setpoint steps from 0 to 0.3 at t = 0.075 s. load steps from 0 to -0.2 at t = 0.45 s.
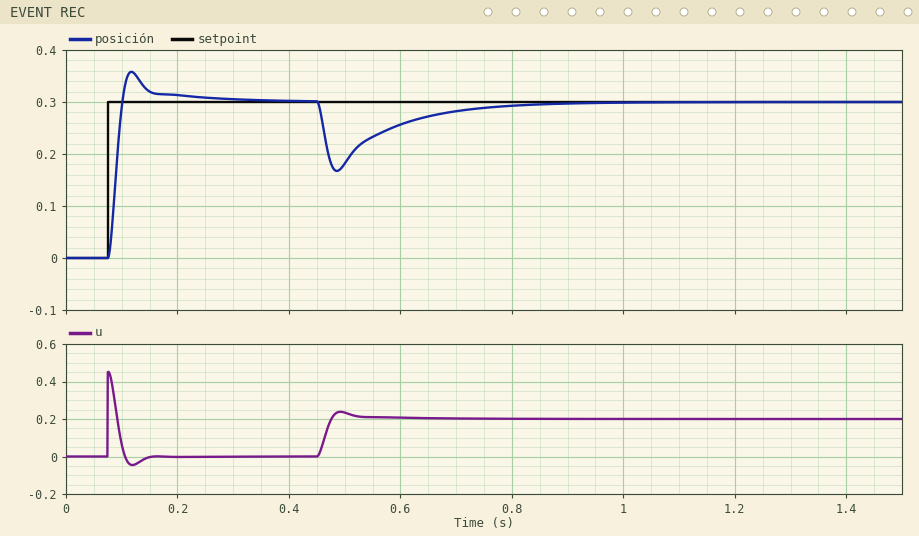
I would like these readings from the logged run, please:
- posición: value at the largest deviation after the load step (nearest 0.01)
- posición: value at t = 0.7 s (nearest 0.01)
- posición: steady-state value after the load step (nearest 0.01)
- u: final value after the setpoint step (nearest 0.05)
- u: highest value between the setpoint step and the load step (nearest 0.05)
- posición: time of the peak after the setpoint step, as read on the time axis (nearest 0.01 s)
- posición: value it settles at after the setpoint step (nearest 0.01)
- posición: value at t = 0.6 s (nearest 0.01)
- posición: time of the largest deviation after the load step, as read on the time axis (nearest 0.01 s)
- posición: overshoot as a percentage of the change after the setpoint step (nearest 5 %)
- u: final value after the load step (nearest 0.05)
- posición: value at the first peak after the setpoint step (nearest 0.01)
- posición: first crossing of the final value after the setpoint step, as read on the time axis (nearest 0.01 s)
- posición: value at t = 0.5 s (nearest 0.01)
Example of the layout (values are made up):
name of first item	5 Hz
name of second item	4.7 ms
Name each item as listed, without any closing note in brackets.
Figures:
posición: value at the largest deviation after the load step	0.17
posición: value at t = 0.7 s	0.28
posición: steady-state value after the load step	0.30
u: final value after the setpoint step	0.00
u: highest value between the setpoint step and the load step	0.45
posición: time of the peak after the setpoint step, as read on the time axis	0.12 s
posición: value it settles at after the setpoint step	0.30
posición: value at t = 0.6 s	0.26
posición: time of the largest deviation after the load step, as read on the time axis	0.49 s
posición: overshoot as a percentage of the change after the setpoint step	20 %
u: final value after the load step	0.20
posición: value at the first peak after the setpoint step	0.36
posición: first crossing of the final value after the setpoint step, as read on the time axis	0.10 s
posición: value at t = 0.5 s	0.18
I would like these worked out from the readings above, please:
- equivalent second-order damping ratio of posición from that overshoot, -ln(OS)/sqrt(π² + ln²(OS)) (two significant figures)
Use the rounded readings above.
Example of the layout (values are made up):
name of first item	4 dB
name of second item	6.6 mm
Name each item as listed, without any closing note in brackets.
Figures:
equivalent second-order damping ratio of posición from that overshoot, -ln(OS)/sqrt(π² + ln²(OS))	0.46
